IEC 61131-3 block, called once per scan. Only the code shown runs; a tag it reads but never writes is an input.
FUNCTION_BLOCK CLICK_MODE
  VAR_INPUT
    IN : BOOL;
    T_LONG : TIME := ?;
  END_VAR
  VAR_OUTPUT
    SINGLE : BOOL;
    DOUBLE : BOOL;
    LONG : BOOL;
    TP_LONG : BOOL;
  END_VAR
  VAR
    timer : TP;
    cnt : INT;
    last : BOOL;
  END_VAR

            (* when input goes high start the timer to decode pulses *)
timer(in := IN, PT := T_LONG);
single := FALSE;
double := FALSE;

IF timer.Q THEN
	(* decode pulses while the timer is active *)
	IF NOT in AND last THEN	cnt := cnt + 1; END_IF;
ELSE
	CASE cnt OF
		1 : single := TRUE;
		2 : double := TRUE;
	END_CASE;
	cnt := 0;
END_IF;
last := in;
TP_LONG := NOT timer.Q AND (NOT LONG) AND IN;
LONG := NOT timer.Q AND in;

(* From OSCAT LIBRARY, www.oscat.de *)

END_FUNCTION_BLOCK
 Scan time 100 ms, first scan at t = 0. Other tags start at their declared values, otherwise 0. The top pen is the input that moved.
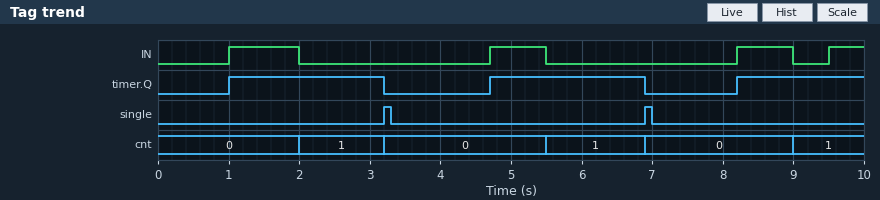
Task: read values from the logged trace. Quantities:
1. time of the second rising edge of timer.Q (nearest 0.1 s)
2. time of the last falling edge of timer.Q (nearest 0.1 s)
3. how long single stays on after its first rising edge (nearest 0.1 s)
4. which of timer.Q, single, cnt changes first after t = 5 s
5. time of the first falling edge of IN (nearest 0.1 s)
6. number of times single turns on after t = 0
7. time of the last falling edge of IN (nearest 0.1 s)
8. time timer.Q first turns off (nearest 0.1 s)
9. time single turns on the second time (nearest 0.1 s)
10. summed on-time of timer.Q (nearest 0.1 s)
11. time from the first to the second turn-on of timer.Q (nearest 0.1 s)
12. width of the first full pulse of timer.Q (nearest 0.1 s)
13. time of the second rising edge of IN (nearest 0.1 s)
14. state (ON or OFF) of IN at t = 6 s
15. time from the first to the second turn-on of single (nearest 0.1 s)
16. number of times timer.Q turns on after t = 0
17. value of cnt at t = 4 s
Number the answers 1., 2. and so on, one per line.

1. 4.7 s
2. 6.9 s
3. 0.1 s
4. cnt
5. 2.0 s
6. 2
7. 9.0 s
8. 3.2 s
9. 6.9 s
10. 6.2 s
11. 3.7 s
12. 2.2 s
13. 4.7 s
14. OFF
15. 3.7 s
16. 3
17. 0
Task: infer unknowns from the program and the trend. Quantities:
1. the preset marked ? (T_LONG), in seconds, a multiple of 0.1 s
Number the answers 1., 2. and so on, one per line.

1. 2.2 s
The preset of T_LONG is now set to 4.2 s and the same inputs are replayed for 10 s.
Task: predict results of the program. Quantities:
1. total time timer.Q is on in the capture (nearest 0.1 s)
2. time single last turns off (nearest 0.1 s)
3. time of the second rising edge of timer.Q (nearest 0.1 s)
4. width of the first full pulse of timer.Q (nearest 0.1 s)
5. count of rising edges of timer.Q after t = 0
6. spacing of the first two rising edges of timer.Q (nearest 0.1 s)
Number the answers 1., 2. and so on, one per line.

1. 6.0 s
2. 5.3 s
3. 8.2 s
4. 4.2 s
5. 2
6. 7.2 s
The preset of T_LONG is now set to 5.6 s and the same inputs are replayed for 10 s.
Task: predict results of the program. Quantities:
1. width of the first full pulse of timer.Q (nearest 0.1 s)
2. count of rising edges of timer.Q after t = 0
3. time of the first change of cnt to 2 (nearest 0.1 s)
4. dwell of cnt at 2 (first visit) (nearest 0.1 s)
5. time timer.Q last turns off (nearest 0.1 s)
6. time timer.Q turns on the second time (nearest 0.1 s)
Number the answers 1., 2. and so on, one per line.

1. 5.6 s
2. 2
3. 5.5 s
4. 1.1 s
5. 6.6 s
6. 8.2 s
